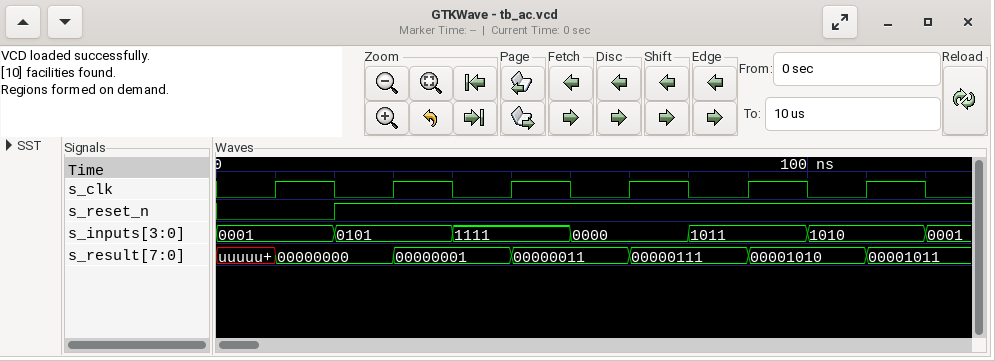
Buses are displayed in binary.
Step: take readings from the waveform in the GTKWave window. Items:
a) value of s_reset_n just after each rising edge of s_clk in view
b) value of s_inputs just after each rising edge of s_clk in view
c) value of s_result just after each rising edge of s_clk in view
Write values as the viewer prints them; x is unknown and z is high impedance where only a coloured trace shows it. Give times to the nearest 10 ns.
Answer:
0 1 1 1 1 1
0001, 0101, 1111, 0000, 1011, 1010
00000000, 00000001, 00000011, 00000111, 00001010, 00001011
